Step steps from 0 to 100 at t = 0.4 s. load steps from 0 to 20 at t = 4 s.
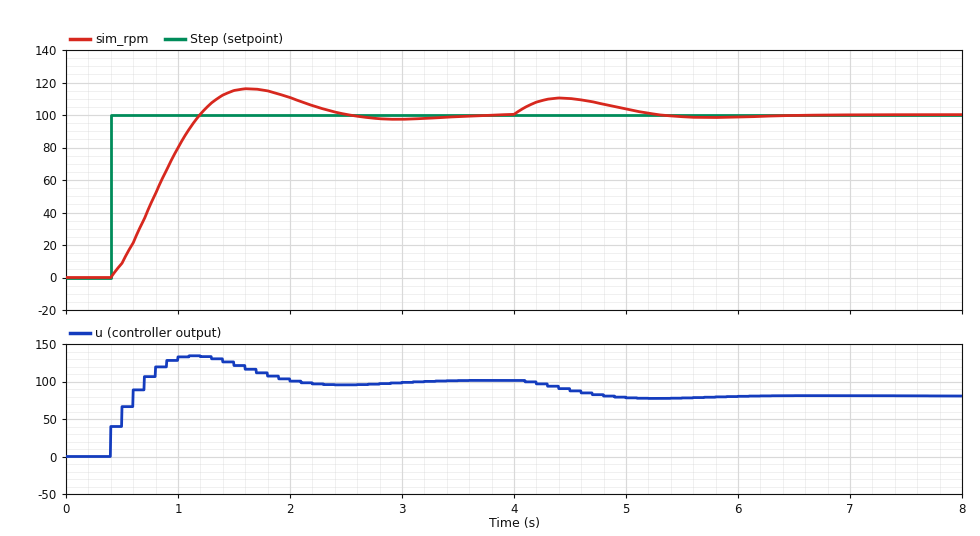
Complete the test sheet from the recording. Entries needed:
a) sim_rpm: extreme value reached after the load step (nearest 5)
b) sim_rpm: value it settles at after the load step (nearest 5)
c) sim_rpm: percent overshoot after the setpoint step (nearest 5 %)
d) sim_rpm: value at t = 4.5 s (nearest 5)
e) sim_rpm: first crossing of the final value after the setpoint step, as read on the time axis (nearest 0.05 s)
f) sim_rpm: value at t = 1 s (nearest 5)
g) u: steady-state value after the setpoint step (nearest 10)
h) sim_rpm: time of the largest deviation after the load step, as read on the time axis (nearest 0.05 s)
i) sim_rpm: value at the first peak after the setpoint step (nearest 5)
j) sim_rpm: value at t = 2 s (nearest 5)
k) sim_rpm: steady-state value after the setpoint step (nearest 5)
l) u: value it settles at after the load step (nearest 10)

110
100
15 %
110
1.20 s
80
100
4.40 s
115
110
100
80
